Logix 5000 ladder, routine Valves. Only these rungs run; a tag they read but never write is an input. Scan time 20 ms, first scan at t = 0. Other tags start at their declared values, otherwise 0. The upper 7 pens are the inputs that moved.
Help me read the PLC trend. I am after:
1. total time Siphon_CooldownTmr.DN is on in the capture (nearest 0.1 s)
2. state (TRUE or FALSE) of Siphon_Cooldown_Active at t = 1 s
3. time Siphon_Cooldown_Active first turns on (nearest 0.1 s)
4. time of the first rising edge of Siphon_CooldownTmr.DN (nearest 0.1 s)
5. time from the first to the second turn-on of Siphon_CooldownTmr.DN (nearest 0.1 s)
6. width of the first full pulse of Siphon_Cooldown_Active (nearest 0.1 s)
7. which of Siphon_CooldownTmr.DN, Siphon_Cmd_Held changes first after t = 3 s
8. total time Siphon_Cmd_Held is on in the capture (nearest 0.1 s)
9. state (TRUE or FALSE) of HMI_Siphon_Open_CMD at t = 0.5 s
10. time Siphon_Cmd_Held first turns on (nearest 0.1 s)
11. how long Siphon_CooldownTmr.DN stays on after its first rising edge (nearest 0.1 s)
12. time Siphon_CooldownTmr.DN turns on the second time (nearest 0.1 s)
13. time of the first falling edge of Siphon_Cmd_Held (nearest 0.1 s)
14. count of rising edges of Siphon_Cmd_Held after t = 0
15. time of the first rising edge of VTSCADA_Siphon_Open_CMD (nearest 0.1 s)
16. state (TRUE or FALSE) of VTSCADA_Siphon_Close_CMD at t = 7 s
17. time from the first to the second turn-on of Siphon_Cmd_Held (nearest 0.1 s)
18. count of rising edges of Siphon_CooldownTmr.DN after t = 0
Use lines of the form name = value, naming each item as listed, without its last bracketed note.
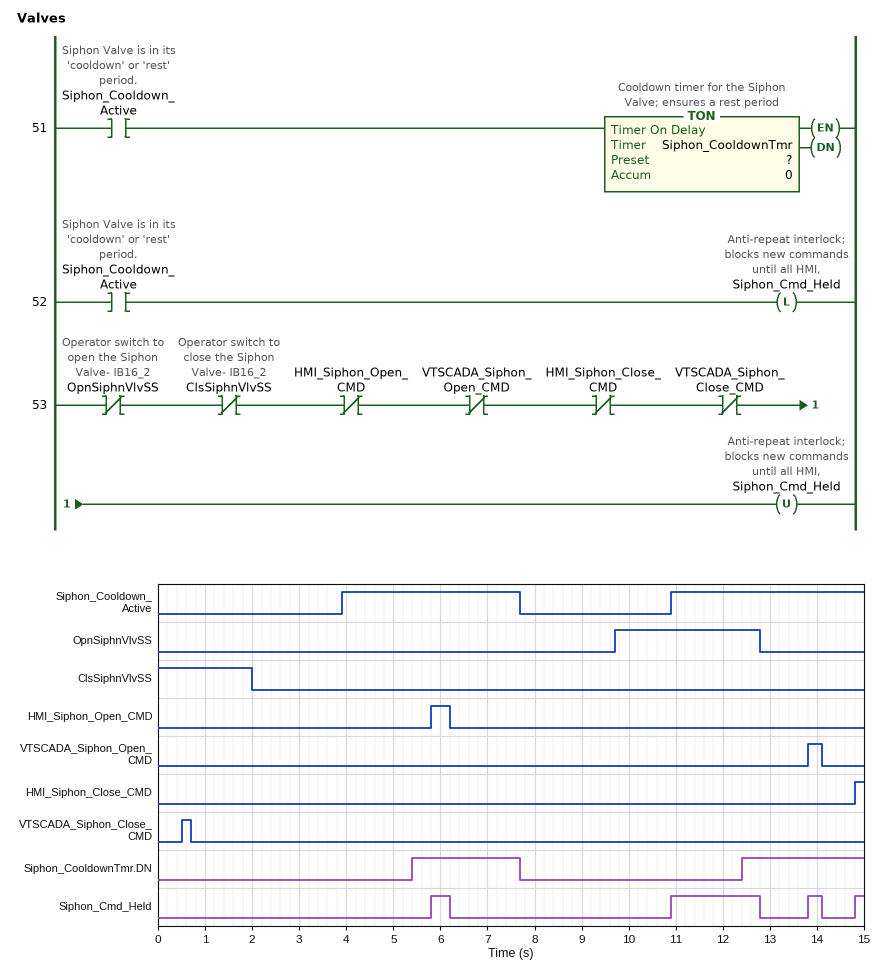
total time Siphon_CooldownTmr.DN is on in the capture = 4.9 s
state (TRUE or FALSE) of Siphon_Cooldown_Active at t = 1 s = FALSE
time Siphon_Cooldown_Active first turns on = 3.9 s
time of the first rising edge of Siphon_CooldownTmr.DN = 5.4 s
time from the first to the second turn-on of Siphon_CooldownTmr.DN = 7.0 s
width of the first full pulse of Siphon_Cooldown_Active = 3.8 s
which of Siphon_CooldownTmr.DN, Siphon_Cmd_Held changes first after t = 3 s = Siphon_CooldownTmr.DN
total time Siphon_Cmd_Held is on in the capture = 2.8 s
state (TRUE or FALSE) of HMI_Siphon_Open_CMD at t = 0.5 s = FALSE
time Siphon_Cmd_Held first turns on = 5.8 s
how long Siphon_CooldownTmr.DN stays on after its first rising edge = 2.3 s
time Siphon_CooldownTmr.DN turns on the second time = 12.4 s
time of the first falling edge of Siphon_Cmd_Held = 6.2 s
count of rising edges of Siphon_Cmd_Held after t = 0 = 4
time of the first rising edge of VTSCADA_Siphon_Open_CMD = 13.8 s
state (TRUE or FALSE) of VTSCADA_Siphon_Close_CMD at t = 7 s = FALSE
time from the first to the second turn-on of Siphon_Cmd_Held = 5.1 s
count of rising edges of Siphon_CooldownTmr.DN after t = 0 = 2
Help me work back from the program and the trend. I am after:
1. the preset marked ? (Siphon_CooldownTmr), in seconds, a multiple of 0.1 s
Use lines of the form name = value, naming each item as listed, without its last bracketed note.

the preset marked ? (Siphon_CooldownTmr), in seconds, a multiple of 0.1 s = 1.5 s
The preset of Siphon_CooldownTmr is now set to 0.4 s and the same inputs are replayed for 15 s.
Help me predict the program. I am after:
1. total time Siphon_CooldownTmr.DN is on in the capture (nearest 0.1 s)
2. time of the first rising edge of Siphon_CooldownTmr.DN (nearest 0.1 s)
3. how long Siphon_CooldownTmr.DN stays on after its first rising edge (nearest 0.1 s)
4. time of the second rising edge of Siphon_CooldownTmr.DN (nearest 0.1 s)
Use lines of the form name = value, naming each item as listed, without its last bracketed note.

total time Siphon_CooldownTmr.DN is on in the capture = 7.1 s
time of the first rising edge of Siphon_CooldownTmr.DN = 4.3 s
how long Siphon_CooldownTmr.DN stays on after its first rising edge = 3.4 s
time of the second rising edge of Siphon_CooldownTmr.DN = 11.3 s
